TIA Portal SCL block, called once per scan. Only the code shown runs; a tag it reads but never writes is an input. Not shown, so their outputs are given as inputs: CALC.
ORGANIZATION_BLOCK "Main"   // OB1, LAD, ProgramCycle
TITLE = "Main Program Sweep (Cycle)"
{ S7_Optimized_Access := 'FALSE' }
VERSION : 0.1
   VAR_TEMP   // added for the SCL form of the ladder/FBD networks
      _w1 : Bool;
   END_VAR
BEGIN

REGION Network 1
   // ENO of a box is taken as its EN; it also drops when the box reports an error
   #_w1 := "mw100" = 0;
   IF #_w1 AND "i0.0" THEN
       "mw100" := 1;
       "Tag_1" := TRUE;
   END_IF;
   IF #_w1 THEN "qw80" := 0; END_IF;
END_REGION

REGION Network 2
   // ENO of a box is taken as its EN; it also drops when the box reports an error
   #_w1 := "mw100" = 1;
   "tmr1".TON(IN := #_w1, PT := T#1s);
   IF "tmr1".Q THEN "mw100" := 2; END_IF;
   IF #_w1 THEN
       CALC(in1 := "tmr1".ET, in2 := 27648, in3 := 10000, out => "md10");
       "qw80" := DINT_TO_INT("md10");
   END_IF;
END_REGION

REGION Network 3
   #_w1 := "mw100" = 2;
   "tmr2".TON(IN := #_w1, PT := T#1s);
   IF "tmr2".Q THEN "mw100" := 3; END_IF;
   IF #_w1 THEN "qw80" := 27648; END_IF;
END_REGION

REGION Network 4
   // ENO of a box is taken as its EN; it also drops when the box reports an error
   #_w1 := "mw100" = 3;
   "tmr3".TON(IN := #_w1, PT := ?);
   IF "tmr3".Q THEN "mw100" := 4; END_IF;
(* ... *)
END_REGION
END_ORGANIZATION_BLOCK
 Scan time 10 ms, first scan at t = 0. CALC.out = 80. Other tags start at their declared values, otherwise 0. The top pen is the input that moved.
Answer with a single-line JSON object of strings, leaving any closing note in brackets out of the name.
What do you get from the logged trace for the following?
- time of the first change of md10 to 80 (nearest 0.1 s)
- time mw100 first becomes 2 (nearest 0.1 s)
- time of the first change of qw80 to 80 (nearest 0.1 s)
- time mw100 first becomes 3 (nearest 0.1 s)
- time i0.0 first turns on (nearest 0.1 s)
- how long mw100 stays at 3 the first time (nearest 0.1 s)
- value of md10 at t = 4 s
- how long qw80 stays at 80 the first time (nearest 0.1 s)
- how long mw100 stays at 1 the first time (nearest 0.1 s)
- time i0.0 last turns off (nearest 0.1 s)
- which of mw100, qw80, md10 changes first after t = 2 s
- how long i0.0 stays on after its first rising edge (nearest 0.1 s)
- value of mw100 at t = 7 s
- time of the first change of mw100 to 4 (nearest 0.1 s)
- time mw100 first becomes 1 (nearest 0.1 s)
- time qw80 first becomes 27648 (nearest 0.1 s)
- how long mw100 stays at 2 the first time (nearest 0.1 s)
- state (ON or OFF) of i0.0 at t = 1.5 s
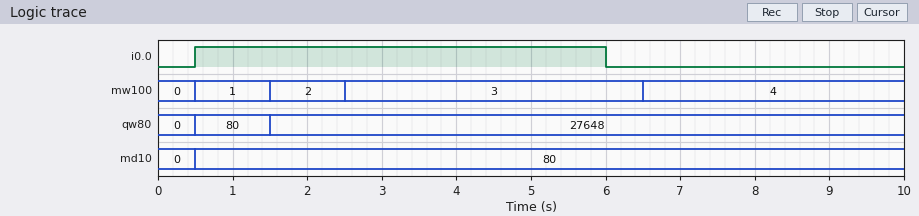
{"time of the first change of md10 to 80": "0.5 s", "time mw100 first becomes 2": "1.5 s", "time of the first change of qw80 to 80": "0.5 s", "time mw100 first becomes 3": "2.5 s", "time i0.0 first turns on": "0.5 s", "how long mw100 stays at 3 the first time": "4.0 s", "value of md10 at t = 4 s": "80", "how long qw80 stays at 80 the first time": "1.0 s", "how long mw100 stays at 1 the first time": "1.0 s", "time i0.0 last turns off": "6.0 s", "which of mw100, qw80, md10 changes first after t = 2 s": "mw100", "how long i0.0 stays on after its first rising edge": "5.5 s", "value of mw100 at t = 7 s": "4", "time of the first change of mw100 to 4": "6.5 s", "time mw100 first becomes 1": "0.5 s", "time qw80 first becomes 27648": "1.5 s", "how long mw100 stays at 2 the first time": "1.0 s", "state (ON or OFF) of i0.0 at t = 1.5 s": "ON"}
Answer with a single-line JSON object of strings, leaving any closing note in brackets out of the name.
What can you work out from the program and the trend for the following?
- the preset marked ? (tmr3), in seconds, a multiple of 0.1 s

{"the preset marked ? (tmr3), in seconds, a multiple of 0.1 s": "4.0 s"}
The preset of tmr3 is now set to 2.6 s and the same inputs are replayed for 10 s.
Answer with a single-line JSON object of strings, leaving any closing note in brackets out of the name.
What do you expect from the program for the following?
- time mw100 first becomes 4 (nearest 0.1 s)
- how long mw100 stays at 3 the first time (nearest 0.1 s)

{"time mw100 first becomes 4": "5.1 s", "how long mw100 stays at 3 the first time": "2.6 s"}
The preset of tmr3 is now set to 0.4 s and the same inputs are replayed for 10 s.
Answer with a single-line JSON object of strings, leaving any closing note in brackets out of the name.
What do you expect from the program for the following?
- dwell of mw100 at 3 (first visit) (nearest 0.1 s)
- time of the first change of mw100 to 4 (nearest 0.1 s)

{"dwell of mw100 at 3 (first visit)": "0.4 s", "time of the first change of mw100 to 4": "2.9 s"}
